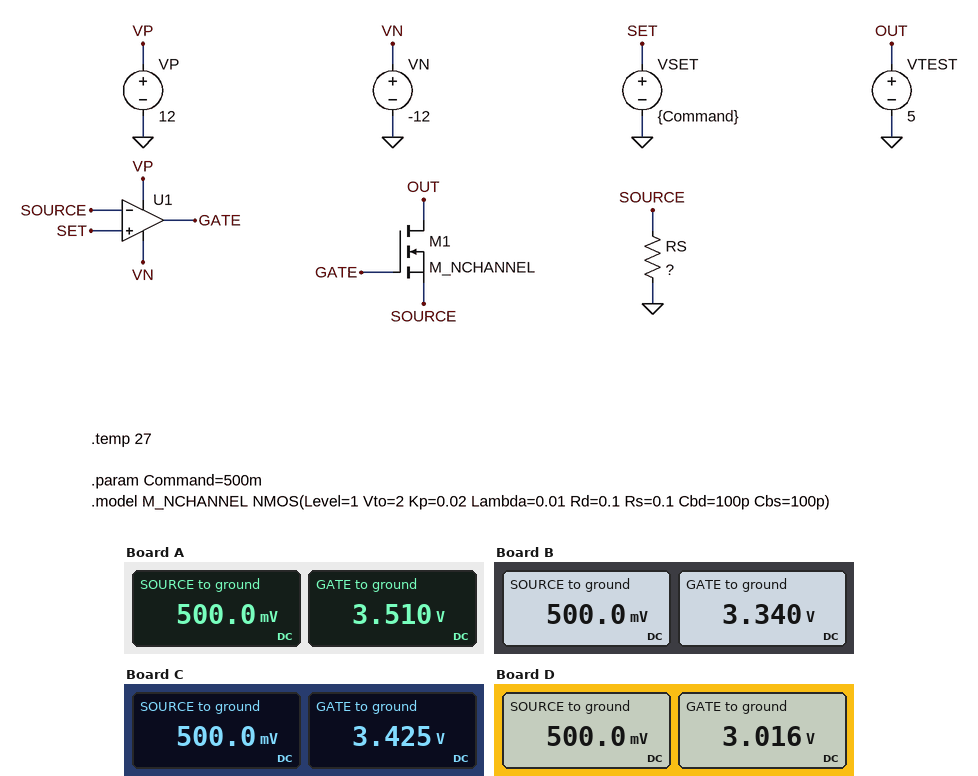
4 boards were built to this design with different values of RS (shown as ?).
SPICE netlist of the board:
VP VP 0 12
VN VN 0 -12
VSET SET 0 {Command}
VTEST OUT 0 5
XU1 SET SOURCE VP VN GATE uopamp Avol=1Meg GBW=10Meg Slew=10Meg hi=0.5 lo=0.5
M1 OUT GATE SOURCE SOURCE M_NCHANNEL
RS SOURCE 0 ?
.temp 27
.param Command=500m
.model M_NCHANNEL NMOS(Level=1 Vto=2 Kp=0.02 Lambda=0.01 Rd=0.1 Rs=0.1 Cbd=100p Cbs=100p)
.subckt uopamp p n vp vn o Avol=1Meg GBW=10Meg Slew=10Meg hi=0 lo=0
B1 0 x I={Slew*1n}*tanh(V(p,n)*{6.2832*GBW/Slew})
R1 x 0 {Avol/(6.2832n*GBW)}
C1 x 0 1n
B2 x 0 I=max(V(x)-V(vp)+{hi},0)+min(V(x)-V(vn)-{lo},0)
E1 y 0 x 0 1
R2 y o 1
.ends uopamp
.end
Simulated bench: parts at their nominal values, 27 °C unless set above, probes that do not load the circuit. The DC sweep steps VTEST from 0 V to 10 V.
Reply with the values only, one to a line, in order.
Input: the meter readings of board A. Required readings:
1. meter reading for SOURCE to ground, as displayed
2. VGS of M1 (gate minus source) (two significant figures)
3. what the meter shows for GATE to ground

500.0 mV
3.0 V
3.510 V
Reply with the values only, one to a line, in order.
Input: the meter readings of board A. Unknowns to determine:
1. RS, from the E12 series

47 Ω
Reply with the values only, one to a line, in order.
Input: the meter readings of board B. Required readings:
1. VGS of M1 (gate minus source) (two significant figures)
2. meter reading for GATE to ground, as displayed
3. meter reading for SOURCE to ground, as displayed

2.8 V
3.340 V
500.0 mV
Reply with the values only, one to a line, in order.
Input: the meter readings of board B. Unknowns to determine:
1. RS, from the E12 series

68 Ω
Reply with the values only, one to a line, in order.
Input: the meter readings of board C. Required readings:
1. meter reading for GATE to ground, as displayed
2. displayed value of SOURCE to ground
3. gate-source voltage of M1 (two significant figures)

3.425 V
500.0 mV
2.9 V
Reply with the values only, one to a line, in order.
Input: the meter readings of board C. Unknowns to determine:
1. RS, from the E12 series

56 Ω
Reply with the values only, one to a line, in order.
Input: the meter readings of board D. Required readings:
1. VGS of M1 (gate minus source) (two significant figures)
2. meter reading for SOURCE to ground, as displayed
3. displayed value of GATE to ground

2.5 V
500.0 mV
3.016 V
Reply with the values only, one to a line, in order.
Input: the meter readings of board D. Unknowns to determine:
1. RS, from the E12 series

180 Ω
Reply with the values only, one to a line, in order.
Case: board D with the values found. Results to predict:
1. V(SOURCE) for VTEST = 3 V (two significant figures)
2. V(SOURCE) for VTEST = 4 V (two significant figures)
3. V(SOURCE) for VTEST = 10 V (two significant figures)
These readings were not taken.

500 mV
500 mV
500 mV
